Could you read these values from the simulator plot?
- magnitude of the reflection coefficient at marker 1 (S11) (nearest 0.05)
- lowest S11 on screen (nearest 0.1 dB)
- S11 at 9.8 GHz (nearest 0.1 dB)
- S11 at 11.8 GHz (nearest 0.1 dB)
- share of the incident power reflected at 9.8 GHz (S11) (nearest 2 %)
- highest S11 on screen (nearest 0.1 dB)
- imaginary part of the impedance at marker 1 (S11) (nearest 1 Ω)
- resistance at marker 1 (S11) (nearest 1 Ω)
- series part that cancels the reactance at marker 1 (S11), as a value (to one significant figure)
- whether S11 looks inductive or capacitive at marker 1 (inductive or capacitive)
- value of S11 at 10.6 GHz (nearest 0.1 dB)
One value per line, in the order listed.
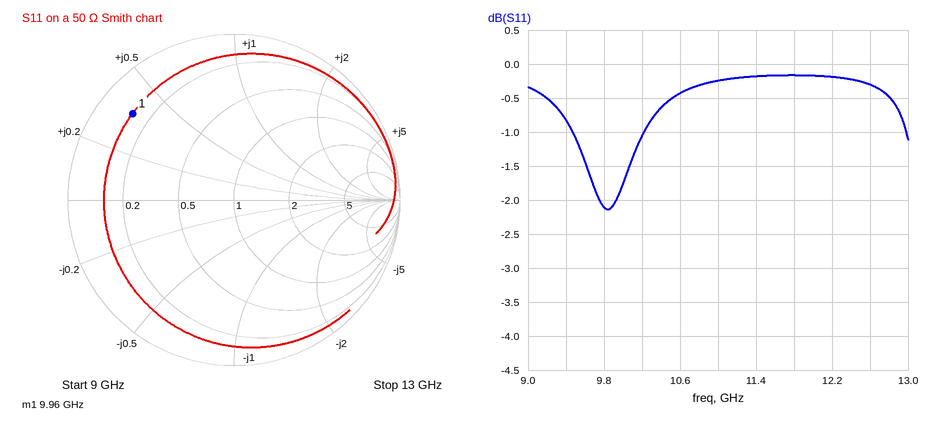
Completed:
0.80
-2.1 dB
-2.1 dB
-0.2 dB
62 %
-0.2 dB
+18 Ω
6 Ω
900 fF
inductive
-0.4 dB
